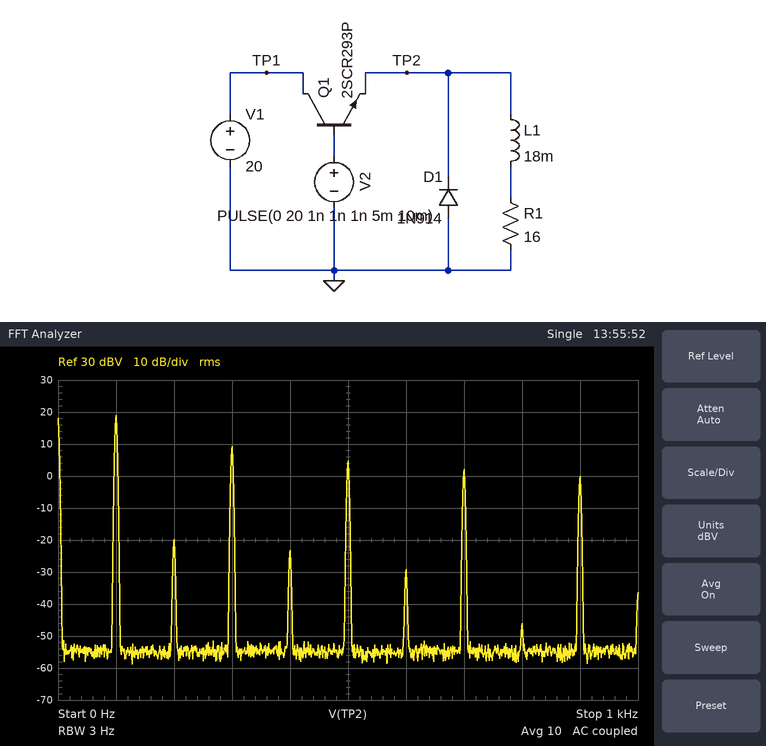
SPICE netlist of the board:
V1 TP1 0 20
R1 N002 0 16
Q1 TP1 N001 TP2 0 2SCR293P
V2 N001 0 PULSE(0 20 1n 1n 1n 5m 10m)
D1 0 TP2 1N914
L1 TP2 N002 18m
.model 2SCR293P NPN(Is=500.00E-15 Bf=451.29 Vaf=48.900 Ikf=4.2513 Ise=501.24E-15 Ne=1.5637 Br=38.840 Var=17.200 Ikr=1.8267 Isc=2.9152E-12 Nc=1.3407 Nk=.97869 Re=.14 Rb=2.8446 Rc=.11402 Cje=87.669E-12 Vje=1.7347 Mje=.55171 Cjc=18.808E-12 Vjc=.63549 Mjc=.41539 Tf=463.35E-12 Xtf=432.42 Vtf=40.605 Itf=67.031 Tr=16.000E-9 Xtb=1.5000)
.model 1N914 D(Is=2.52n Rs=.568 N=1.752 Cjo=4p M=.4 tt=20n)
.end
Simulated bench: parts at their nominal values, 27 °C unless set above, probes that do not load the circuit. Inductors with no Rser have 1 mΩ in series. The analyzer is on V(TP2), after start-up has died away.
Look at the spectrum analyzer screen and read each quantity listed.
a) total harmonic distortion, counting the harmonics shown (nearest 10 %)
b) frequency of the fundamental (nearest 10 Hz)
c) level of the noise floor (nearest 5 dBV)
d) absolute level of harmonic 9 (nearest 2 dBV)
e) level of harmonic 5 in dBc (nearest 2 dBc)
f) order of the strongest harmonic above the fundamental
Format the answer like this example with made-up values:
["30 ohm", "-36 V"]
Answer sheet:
["40 %", "100 Hz", "-55 dBV", "0 dBV", "-14 dBc", "3"]
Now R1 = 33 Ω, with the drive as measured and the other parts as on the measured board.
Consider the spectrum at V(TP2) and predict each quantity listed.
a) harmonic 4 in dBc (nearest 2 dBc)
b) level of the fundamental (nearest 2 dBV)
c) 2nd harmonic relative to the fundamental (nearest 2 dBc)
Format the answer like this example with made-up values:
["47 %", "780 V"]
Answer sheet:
["-44 dBc", "18 dBV", "-36 dBc"]
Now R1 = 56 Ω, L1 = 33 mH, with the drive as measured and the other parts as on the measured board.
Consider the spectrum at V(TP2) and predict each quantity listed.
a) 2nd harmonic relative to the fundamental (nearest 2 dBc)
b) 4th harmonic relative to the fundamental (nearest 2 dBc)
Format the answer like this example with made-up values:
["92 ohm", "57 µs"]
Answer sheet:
["-36 dBc", "-46 dBc"]
